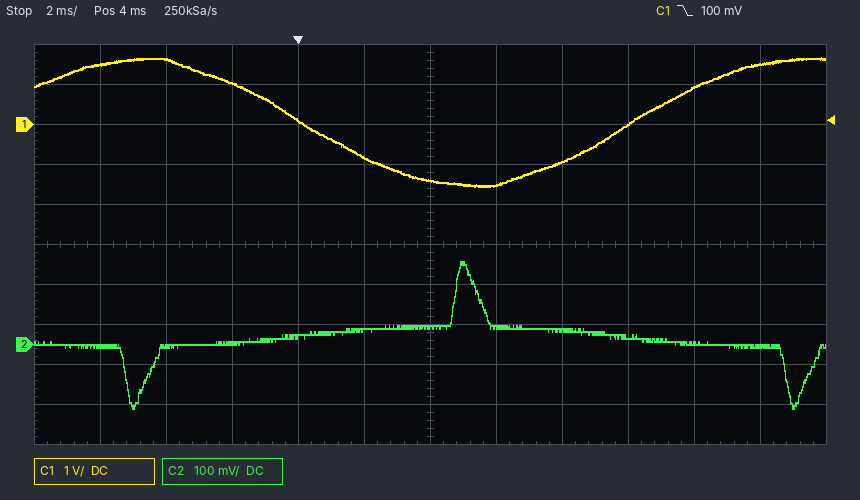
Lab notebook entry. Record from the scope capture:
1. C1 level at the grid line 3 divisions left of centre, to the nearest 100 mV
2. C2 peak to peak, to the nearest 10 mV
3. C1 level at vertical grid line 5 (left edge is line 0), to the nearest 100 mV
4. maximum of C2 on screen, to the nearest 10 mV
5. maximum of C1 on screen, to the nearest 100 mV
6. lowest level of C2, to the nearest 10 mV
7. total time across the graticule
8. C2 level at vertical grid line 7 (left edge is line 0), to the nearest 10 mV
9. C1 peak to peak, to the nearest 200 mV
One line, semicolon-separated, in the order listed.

1.0 V; 370 mV; -800 mV; 210 mV; 1.7 V; -160 mV; 24 ms; 40 mV; 3.2 V
